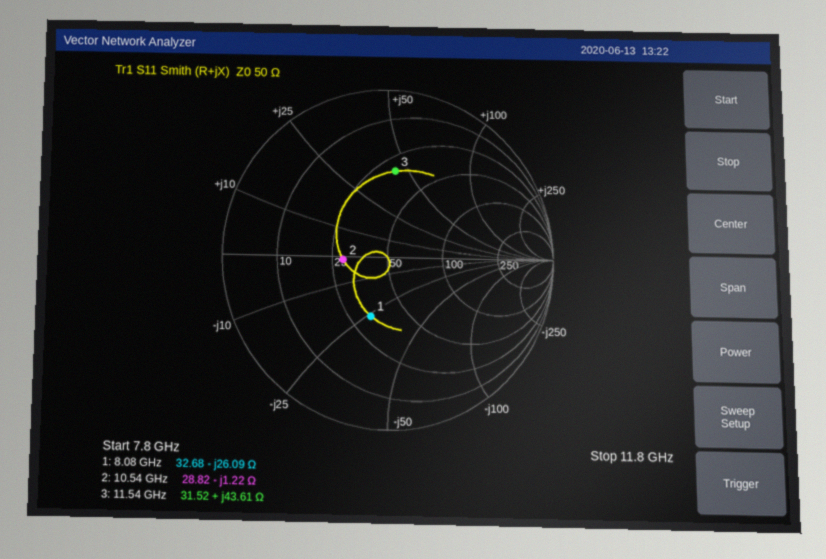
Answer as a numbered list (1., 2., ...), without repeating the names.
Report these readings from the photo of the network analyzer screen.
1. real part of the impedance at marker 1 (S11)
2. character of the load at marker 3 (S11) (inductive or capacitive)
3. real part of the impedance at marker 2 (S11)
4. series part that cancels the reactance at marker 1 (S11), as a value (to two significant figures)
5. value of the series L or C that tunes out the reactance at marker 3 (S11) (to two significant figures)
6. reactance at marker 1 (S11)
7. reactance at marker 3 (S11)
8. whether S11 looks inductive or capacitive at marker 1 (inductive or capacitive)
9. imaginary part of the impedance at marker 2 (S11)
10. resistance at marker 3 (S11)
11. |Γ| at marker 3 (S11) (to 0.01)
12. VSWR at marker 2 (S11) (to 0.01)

1. 32.68 Ω
2. inductive
3. 28.82 Ω
4. 510 pH
5. 320 fF
6. -26.09 Ω
7. +43.61 Ω
8. capacitive
9. -1.22 Ω
10. 31.52 Ω
11. 0.51
12. 1.74
